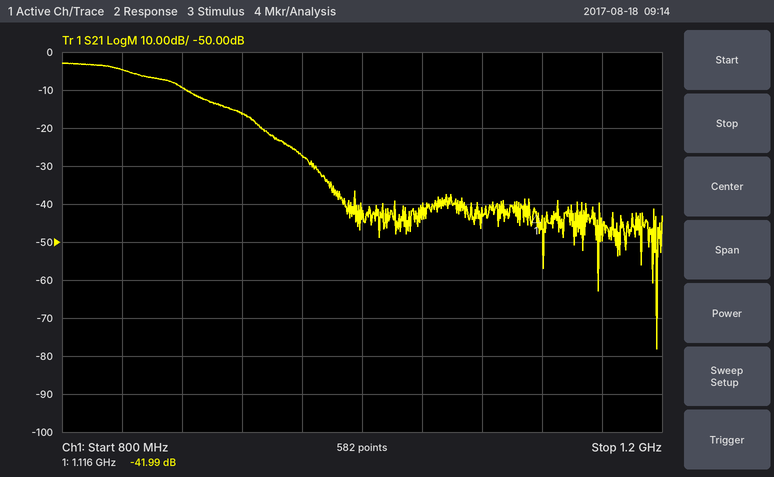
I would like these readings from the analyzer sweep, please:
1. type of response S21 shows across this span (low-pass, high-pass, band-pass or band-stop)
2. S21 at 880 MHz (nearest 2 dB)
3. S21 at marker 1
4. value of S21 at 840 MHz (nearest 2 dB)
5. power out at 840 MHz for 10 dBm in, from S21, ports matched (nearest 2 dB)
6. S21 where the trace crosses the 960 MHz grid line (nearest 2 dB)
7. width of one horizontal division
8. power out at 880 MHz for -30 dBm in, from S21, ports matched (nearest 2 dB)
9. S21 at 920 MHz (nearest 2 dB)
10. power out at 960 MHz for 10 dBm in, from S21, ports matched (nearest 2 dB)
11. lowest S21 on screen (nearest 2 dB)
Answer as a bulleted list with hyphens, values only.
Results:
- low-pass
- -10 dB
- -41.99 dB
- -4 dB
- 6 dBm
- -28 dB
- 40 MHz
- -40 dBm
- -16 dB
- -18 dBm
- -78 dB
